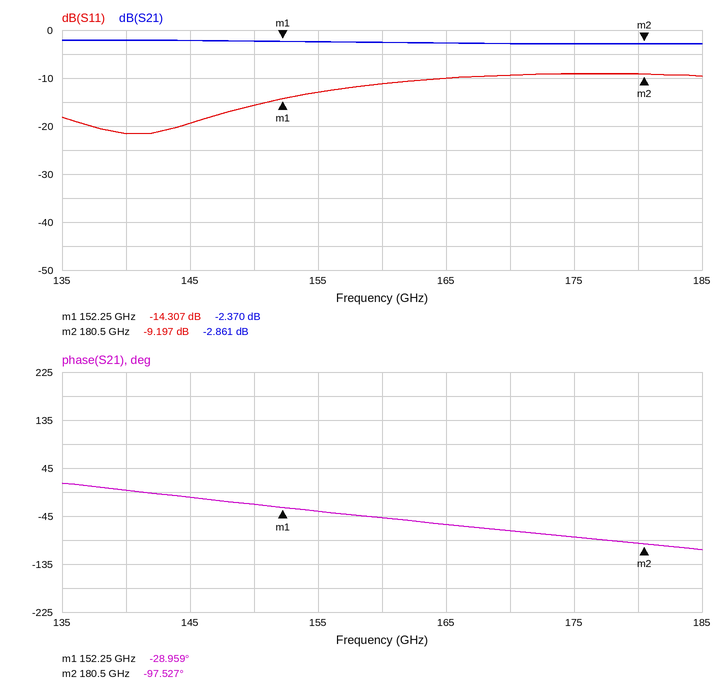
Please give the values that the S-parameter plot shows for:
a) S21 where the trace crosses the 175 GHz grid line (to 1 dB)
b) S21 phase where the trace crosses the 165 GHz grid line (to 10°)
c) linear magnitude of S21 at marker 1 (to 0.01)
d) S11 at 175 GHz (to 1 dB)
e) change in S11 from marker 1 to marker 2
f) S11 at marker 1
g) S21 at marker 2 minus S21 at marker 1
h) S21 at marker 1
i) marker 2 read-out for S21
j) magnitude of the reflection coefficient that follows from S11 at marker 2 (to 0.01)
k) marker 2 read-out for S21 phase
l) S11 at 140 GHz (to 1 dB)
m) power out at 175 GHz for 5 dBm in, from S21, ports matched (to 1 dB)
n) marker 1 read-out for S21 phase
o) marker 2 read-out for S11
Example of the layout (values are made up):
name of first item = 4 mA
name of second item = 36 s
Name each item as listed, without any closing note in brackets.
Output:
S21 where the trace crosses the 175 GHz grid line = -3 dB
S21 phase where the trace crosses the 165 GHz grid line = -60°
linear magnitude of S21 at marker 1 = 0.76
S11 at 175 GHz = -9 dB
change in S11 from marker 1 to marker 2 = 5.110 dB
S11 at marker 1 = -14.307 dB
S21 at marker 2 minus S21 at marker 1 = -0.491 dB
S21 at marker 1 = -2.370 dB
marker 2 read-out for S21 = -2.861 dB
magnitude of the reflection coefficient that follows from S11 at marker 2 = 0.35
marker 2 read-out for S21 phase = -97.527°
S11 at 140 GHz = -22 dB
power out at 175 GHz for 5 dBm in, from S21, ports matched = 2 dBm
marker 1 read-out for S21 phase = -28.959°
marker 2 read-out for S11 = -9.197 dB
